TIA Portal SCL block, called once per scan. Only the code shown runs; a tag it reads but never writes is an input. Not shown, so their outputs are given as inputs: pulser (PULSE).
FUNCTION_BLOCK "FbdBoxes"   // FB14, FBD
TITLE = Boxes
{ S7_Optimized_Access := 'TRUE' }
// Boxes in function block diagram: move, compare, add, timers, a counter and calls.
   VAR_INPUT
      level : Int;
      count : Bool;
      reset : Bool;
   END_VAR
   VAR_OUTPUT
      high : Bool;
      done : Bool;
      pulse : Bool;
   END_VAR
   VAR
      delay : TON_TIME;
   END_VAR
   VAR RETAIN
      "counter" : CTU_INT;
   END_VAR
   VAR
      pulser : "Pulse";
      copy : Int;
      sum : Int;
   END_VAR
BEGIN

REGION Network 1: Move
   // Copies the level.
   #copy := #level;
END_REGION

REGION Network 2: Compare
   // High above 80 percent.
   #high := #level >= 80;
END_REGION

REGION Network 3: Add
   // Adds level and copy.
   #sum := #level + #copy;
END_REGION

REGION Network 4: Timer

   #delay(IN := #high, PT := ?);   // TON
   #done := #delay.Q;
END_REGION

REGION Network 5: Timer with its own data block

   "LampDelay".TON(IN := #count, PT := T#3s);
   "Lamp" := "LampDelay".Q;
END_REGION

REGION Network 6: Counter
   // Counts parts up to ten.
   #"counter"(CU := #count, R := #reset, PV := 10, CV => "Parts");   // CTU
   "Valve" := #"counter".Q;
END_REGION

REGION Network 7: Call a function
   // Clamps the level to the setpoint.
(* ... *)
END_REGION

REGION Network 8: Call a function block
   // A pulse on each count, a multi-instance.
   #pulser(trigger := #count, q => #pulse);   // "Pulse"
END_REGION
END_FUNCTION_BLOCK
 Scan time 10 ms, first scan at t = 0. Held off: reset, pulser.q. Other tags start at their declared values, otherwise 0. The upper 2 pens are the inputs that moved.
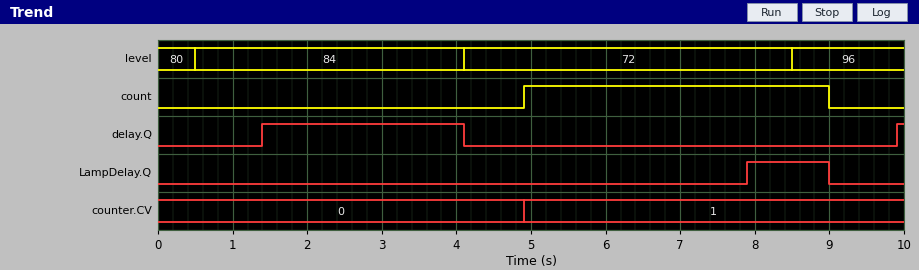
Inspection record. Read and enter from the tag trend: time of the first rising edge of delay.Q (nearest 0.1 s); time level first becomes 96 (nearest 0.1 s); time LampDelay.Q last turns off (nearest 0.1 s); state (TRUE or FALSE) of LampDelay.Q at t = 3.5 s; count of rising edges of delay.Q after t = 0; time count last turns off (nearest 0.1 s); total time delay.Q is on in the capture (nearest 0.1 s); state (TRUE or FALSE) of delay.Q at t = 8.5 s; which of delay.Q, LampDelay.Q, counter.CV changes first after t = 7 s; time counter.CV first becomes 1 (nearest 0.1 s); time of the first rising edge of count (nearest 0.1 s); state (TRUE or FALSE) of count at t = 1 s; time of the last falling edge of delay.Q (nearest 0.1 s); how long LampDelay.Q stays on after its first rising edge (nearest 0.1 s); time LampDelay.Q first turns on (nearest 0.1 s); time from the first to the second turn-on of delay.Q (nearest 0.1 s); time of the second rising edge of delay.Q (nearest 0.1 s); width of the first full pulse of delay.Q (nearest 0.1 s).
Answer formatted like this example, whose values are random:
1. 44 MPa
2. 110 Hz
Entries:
1. 1.4 s
2. 8.5 s
3. 9.0 s
4. FALSE
5. 2
6. 9.0 s
7. 2.8 s
8. FALSE
9. LampDelay.Q
10. 4.9 s
11. 4.9 s
12. FALSE
13. 4.1 s
14. 1.1 s
15. 7.9 s
16. 8.5 s
17. 9.9 s
18. 2.7 s
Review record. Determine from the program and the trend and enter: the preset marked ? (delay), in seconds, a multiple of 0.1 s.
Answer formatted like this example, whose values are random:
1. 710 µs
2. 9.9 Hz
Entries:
1. 1.4 s
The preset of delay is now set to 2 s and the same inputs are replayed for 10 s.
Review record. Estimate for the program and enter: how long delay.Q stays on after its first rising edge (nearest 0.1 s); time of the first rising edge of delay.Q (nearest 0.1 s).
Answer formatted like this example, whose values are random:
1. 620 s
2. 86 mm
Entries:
1. 2.1 s
2. 2.0 s
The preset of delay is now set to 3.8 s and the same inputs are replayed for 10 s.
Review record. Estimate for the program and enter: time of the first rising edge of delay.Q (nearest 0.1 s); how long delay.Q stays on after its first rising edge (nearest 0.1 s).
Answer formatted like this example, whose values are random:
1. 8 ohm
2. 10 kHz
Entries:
1. 3.8 s
2. 0.3 s
